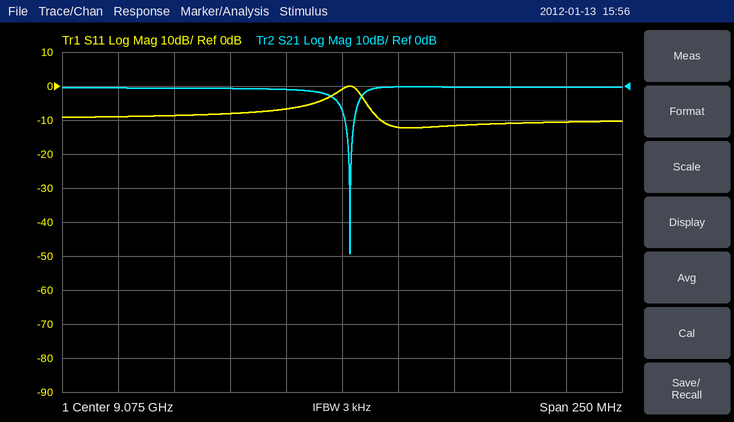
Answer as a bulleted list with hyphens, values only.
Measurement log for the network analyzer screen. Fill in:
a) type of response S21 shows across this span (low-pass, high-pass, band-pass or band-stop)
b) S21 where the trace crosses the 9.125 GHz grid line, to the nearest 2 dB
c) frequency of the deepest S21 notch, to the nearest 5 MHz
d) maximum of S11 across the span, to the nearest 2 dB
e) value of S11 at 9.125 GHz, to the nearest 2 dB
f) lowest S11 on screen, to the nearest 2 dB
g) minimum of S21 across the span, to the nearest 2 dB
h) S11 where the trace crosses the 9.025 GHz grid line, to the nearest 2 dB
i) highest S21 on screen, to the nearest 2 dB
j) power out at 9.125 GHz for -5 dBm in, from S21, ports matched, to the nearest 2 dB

- band-stop
- 0 dB
- 9.080 GHz
- 0 dB
- -12 dB
- -12 dB
- -50 dB
- -8 dB
- 0 dB
- -6 dBm
